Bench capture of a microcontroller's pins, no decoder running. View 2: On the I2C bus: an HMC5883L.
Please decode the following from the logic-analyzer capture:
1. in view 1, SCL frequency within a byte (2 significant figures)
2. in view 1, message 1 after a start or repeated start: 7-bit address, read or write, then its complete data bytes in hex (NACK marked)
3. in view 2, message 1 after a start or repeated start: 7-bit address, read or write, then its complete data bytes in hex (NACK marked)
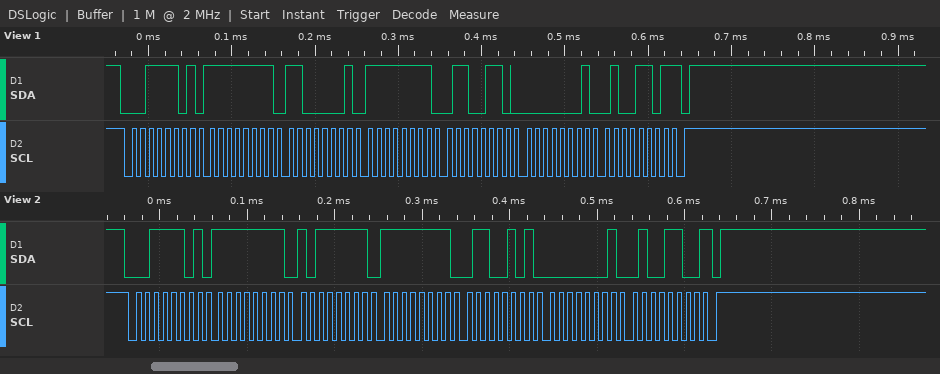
100 kHz
0x1E read: FF C1 FF 66 01 4D NACK
0x1E read: FF BF FF 65 01 4C NACK
